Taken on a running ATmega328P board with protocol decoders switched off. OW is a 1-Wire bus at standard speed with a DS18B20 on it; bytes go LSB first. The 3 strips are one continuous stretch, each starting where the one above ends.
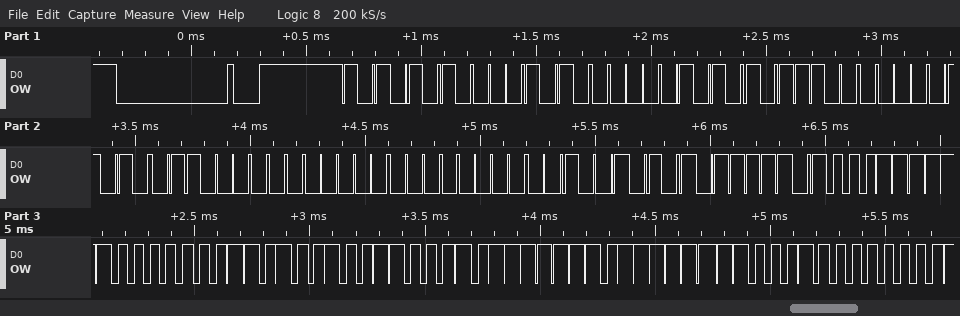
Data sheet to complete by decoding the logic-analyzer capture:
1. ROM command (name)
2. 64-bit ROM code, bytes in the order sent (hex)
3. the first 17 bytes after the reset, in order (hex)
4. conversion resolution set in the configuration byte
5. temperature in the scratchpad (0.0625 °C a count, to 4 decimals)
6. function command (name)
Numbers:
Match ROM
28 50 1D 50 06 00 00 A9
55 28 50 1D 50 06 00 00 A9 BE F8 01 4B 46 7F FF 08
12 bits
31.5000 °C
Read Scratchpad
